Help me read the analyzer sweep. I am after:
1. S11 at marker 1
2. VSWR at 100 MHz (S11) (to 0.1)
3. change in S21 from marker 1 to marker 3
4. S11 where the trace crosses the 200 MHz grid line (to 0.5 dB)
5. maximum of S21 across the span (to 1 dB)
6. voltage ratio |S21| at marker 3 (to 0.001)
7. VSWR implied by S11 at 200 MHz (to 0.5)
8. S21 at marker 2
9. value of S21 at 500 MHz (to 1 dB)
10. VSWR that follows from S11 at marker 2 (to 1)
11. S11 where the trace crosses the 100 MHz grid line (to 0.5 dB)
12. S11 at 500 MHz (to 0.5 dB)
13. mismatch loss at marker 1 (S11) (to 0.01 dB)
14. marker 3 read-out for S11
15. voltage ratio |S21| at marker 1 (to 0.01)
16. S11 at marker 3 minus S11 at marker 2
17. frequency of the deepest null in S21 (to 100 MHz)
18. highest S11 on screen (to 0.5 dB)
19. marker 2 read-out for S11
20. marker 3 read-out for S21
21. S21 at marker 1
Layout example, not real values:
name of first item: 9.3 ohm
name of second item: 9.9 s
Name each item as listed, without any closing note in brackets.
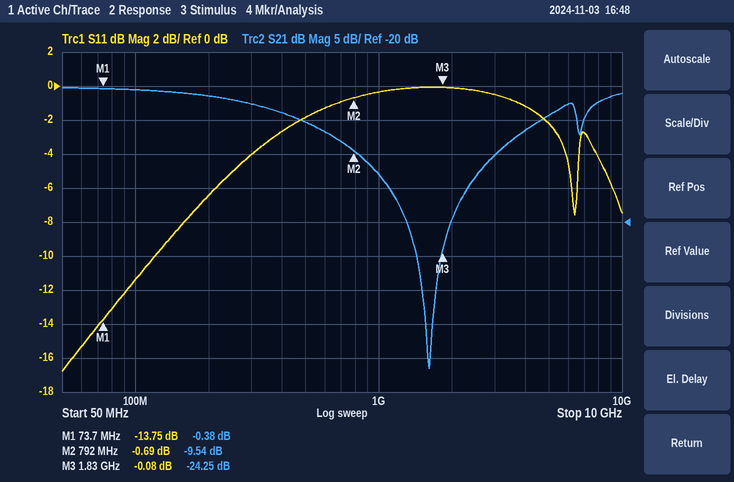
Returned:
S11 at marker 1: -13.75 dB
VSWR at 100 MHz (S11): 1.7
change in S21 from marker 1 to marker 3: -23.87 dB
S11 where the trace crosses the 200 MHz grid line: -6.5 dB
maximum of S21 across the span: 0 dB
voltage ratio |S21| at marker 3: 0.061
VSWR implied by S11 at 200 MHz: 3.0
S21 at marker 2: -9.54 dB
value of S21 at 500 MHz: -5 dB
VSWR that follows from S11 at marker 2: 25
S11 where the trace crosses the 100 MHz grid line: -11.5 dB
S11 at 500 MHz: -2.0 dB
mismatch loss at marker 1 (S11): 0.19 dB
marker 3 read-out for S11: -0.08 dB
voltage ratio |S21| at marker 1: 0.96
S11 at marker 3 minus S11 at marker 2: 0.61 dB
frequency of the deepest null in S21: 1.6 GHz
highest S11 on screen: 0.0 dB
marker 2 read-out for S11: -0.69 dB
marker 3 read-out for S21: -24.25 dB
S21 at marker 1: -0.38 dB
